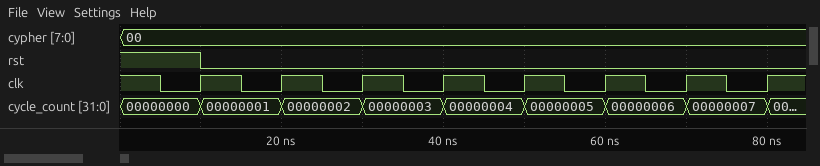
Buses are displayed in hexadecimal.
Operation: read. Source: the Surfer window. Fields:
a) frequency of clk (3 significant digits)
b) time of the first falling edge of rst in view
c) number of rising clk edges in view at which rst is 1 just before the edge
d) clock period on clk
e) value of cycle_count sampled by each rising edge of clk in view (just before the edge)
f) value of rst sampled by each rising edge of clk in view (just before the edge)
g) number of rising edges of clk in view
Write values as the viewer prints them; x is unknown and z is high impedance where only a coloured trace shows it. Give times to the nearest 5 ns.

100 MHz
10 ns
1
10 ns
00000000, 00000001, 00000002, 00000003, 00000004, 00000005, 00000006, 00000007
1 0 0 0 0 0 0 0
8
